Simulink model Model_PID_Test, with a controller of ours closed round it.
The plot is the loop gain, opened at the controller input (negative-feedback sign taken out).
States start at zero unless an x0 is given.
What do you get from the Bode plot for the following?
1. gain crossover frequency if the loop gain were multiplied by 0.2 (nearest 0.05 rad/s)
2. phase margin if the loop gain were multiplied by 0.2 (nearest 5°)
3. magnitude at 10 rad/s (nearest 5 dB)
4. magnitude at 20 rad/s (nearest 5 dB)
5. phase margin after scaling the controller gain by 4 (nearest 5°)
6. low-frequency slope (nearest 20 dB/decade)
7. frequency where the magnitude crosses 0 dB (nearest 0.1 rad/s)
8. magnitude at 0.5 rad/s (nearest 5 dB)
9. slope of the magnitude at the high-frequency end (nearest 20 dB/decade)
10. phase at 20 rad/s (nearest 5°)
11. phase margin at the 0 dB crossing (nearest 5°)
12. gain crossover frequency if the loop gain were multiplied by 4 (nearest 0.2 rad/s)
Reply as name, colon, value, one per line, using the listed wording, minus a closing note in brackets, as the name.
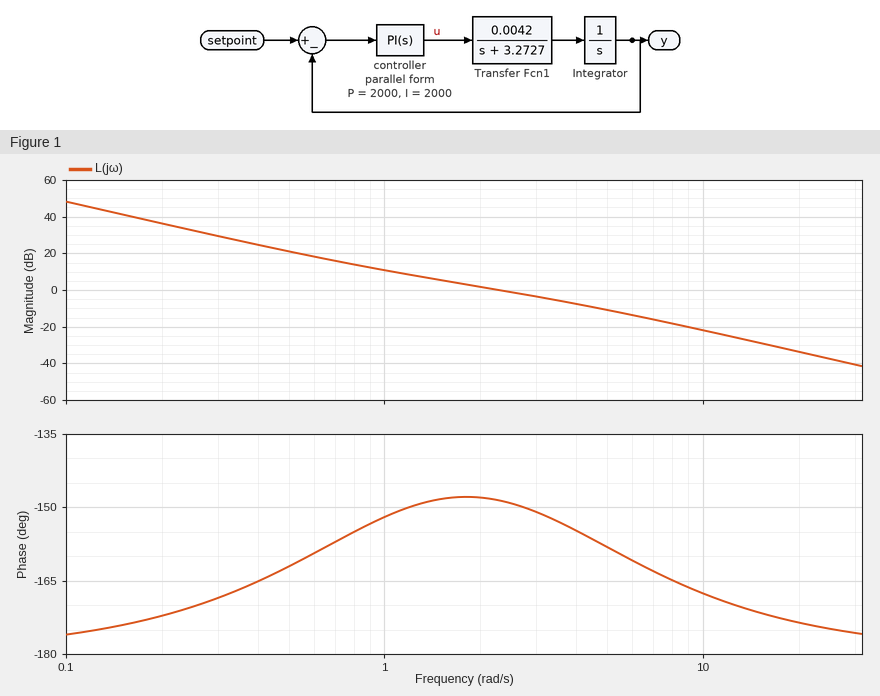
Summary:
gain crossover frequency if the loop gain were multiplied by 0.2: 0.80 rad/s
phase margin if the loop gain were multiplied by 0.2: 25°
magnitude at 10 rad/s: -20 dB
magnitude at 20 rad/s: -35 dB
phase margin after scaling the controller gain by 4: 20°
low-frequency slope: -40 dB/decade
frequency where the magnitude crosses 0 dB: 2.3 rad/s
magnitude at 0.5 rad/s: 20 dB
slope of the magnitude at the high-frequency end: -40 dB/decade
phase at 20 rad/s: -175°
phase margin at the 0 dB crossing: 30°
gain crossover frequency if the loop gain were multiplied by 4: 5.4 rad/s
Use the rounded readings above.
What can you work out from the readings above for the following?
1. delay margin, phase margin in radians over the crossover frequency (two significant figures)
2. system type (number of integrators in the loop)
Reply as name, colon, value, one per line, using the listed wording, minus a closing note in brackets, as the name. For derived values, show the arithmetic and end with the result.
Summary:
delay margin, phase margin in radians over the crossover frequency: 30 × π / 180 / 2.3 = 0.23 s
system type: 2
